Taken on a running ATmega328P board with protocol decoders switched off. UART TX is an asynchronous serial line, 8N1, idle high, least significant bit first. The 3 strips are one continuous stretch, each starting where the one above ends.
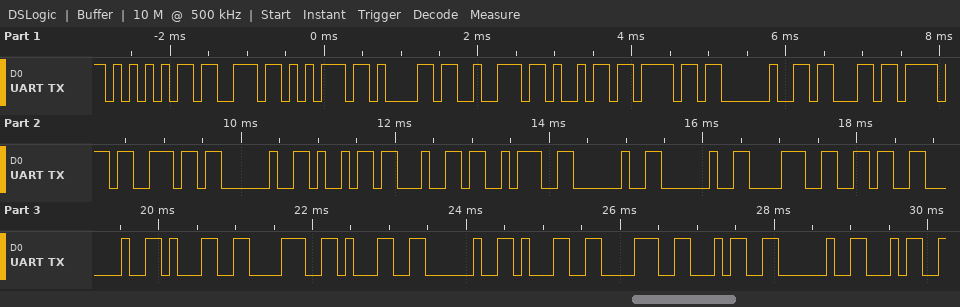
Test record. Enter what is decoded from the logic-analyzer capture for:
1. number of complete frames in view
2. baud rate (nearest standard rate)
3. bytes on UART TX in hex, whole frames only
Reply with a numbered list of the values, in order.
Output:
1. 29
2. 9600 baud
3. 0x55 0x73 0x75 0x61 0x72 0x69 0x6F 0x20 0x63 0x6F 0x6E 0x20 0x69 0x64 0x3A 0x20 0x20 0x38 0x36 0x20 0x31 0x38 0x31 0x20 0x31 0x38 0x34 0x20 0x34
